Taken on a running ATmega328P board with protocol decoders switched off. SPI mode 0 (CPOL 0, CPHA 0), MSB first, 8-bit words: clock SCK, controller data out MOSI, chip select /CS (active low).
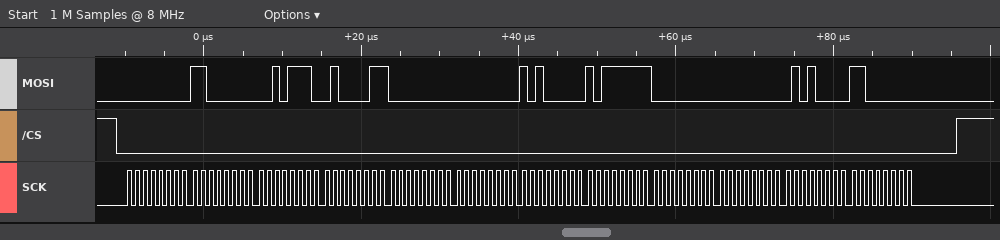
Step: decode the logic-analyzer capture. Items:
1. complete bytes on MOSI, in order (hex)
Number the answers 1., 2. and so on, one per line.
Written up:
1. 0x00 0xC0 0x2E 0x43 0x00 0x00 0xA0 0xBF 0x00 0x00 0x50 0xC0
